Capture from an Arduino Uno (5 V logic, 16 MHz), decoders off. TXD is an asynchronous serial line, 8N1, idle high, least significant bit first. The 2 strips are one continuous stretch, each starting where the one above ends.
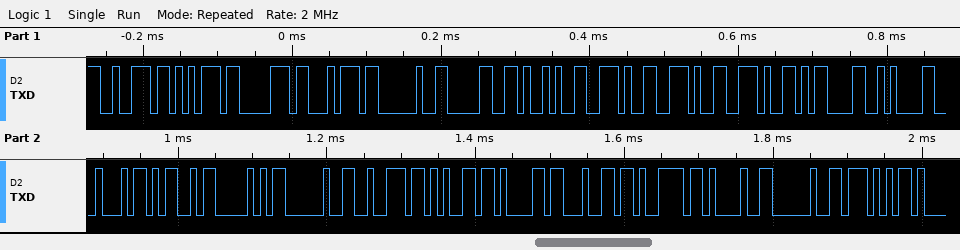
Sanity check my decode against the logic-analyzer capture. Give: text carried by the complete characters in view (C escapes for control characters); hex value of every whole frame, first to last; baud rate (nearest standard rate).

"rupt 0)...\r\nDMP ready! W"
72 75 70 74 20 30 29 2E 2E 2E 0D 0A 44 4D 50 20 72 65 61 64 79 21 20 57
115200 baud
